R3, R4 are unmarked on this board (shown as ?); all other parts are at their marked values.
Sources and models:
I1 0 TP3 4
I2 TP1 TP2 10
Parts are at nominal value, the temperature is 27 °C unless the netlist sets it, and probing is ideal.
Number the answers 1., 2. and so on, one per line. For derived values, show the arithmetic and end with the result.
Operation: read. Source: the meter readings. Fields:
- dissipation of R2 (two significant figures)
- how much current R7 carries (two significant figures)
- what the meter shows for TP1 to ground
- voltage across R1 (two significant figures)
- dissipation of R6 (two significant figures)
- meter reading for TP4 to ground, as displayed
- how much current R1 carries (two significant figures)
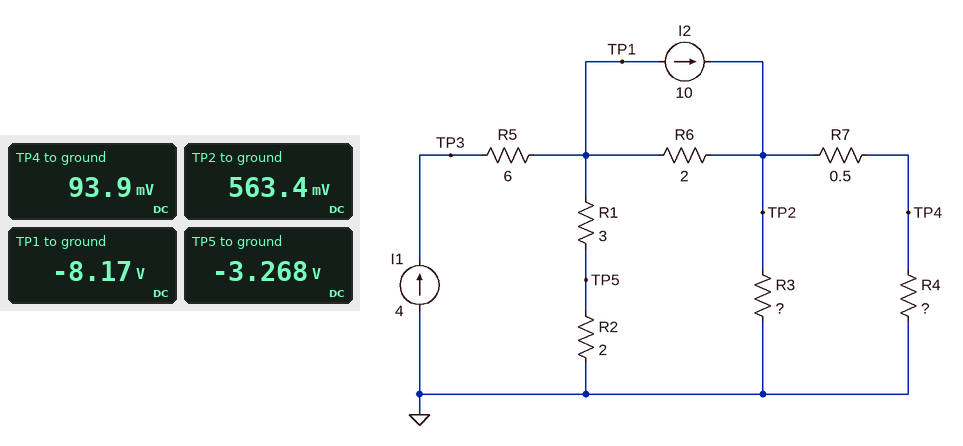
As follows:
1. (0 V - (-3.268 V))^2 / 2 Ω = 5.3 W
2. (563.4 mV - 93.9 mV) / 500 mΩ = 940 mA
3. -8.17 V
4. -3.268 V - (-8.17 V) = 4.9 V
5. (563.4 mV - (-8.17 V))^2 / 2 Ω = 38 W
6. 93.9 mV
7. (-3.268 V - (-8.17 V)) / 3 Ω = 1.6 A
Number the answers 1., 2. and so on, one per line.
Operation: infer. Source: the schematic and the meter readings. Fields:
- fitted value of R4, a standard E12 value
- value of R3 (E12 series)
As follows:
1. 0.1 Ω
2. 0.12 Ω
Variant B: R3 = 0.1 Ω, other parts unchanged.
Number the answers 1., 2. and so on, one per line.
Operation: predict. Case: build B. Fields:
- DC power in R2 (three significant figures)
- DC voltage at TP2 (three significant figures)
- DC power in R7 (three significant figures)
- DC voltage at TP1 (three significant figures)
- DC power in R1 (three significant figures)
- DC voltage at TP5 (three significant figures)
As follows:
1. 5.41 W
2. 484 mV
3. 325 mW
4. -8.23 V
5. 8.12 W
6. -3.29 V
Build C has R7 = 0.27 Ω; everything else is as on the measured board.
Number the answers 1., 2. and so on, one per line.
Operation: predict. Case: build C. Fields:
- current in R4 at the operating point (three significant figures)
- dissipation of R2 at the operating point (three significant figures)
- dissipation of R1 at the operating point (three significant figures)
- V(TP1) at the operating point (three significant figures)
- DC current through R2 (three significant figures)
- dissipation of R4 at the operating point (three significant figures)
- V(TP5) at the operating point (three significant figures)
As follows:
1. 1.38 A
2. 5.39 W
3. 8.08 W
4. -8.21 V
5. 1.64 A
6. 191 mW
7. -3.28 V
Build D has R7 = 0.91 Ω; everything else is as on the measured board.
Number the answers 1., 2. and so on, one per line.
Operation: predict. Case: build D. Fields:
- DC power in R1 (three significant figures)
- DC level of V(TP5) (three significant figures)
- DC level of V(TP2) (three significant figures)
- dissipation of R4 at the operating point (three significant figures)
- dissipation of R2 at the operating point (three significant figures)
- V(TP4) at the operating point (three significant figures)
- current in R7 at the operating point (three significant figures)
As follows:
1. 7.95 W
2. -3.26 V
3. 604 mV
4. 35.7 mW
5. 5.30 W
6. 59.8 mV
7. 598 mA
